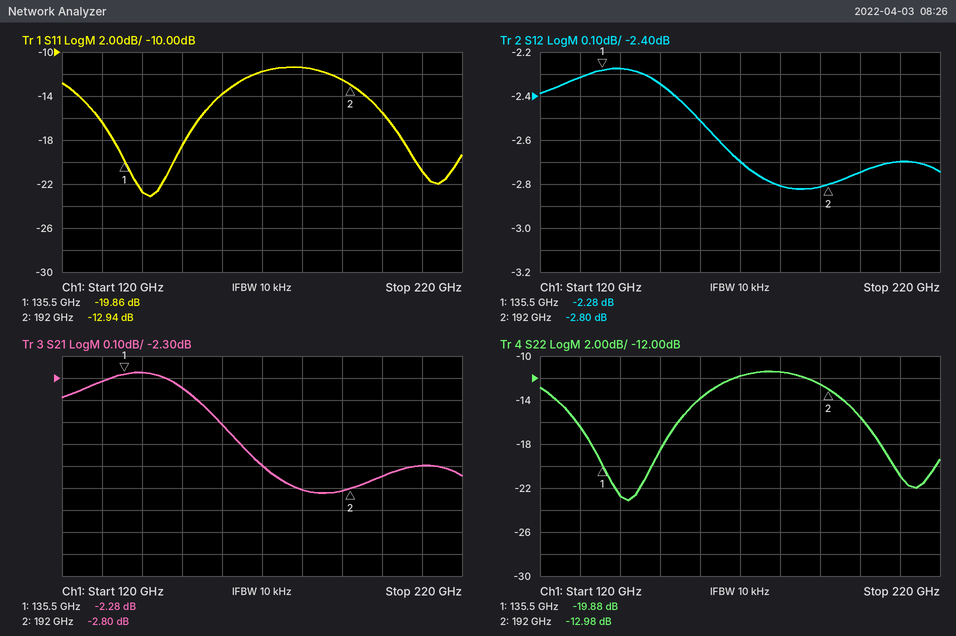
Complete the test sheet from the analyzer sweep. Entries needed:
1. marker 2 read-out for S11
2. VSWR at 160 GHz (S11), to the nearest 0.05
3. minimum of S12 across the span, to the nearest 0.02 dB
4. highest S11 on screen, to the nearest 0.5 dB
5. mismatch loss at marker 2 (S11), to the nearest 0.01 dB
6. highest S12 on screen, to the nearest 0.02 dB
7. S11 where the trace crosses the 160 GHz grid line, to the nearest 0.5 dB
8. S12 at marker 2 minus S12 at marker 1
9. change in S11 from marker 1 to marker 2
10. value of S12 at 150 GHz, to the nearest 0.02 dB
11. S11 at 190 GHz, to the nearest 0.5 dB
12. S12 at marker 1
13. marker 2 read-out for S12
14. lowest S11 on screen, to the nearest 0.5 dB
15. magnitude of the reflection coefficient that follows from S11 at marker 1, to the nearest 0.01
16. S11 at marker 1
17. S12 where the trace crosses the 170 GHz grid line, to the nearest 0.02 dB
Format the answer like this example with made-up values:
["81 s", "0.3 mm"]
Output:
["-12.94 dB", "1.50", "-2.82 dB", "-11.5 dB", "0.23 dB", "-2.28 dB", "-14.0 dB", "-0.52 dB", "6.92 dB", "-2.34 dB", "-12.5 dB", "-2.28 dB", "-2.80 dB", "-23.0 dB", "0.10", "-19.86 dB", "-2.70 dB"]
